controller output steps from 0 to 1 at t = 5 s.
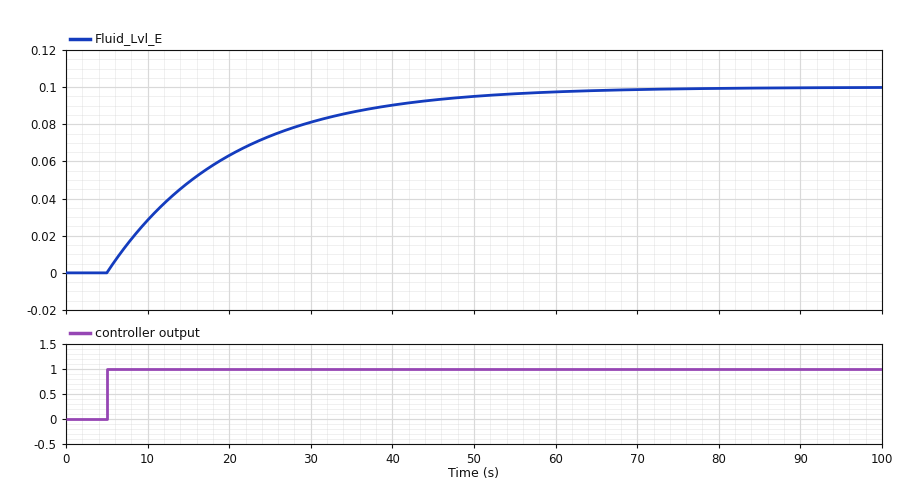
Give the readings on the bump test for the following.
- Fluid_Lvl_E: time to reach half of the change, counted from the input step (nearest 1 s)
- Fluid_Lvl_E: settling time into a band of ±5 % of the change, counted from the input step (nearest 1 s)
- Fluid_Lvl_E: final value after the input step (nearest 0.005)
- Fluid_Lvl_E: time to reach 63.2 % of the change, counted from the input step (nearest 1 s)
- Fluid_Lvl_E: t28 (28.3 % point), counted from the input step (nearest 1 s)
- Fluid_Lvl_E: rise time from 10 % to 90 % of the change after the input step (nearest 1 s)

10 s
45 s
0.100
15 s
5 s
33 s
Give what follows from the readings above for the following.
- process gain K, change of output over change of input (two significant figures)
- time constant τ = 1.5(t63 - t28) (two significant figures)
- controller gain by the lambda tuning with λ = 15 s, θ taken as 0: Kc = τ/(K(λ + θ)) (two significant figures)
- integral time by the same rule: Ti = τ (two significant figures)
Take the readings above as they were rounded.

0.10
15 s
10
15 s
